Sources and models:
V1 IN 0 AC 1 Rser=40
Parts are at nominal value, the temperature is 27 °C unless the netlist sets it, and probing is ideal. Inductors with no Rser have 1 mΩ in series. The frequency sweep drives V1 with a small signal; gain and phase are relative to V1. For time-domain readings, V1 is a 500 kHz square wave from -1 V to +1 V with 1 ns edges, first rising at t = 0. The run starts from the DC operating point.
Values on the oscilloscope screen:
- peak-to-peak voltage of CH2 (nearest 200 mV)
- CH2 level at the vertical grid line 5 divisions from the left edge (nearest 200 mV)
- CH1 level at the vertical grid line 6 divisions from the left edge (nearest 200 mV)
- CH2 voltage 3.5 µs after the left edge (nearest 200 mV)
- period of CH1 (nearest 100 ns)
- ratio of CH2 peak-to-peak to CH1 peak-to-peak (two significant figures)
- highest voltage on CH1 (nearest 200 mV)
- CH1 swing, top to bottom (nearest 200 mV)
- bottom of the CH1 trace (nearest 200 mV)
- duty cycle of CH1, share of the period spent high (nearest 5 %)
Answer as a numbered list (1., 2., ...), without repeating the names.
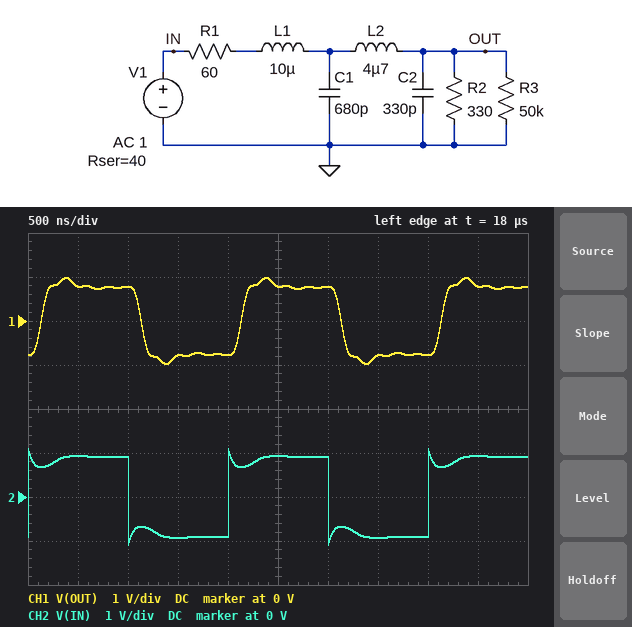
1. 2.2 V
2. 1.0 V
3. 800 mV
4. -1.0 V
5. 2.0 µs
6. 1.1
7. 1.0 V
8. 2.0 V
9. -1.0 V
10. 50 %
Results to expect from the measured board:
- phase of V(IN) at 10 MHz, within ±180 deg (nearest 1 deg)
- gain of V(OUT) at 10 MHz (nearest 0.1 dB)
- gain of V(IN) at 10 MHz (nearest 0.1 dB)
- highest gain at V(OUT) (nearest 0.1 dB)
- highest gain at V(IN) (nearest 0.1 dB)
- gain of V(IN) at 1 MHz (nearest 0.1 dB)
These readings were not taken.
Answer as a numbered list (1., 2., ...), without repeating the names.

1. 4 deg
2. -41.8 dB
3. -0.1 dB
4. -1.5 dB
5. 0 dB
6. -2.0 dB
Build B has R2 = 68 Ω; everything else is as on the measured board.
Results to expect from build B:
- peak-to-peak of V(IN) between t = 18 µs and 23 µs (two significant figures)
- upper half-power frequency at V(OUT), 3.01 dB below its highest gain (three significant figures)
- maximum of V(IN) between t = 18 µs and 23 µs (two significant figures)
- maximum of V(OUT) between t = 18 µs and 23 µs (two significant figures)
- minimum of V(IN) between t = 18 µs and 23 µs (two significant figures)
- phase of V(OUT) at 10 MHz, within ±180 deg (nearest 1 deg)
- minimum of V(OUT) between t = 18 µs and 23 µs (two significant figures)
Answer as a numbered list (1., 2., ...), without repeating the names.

1. 2.5 V
2. 3.84 MHz
3. 1.2 V
4. 440 mV
5. -1.2 V
6. 50 deg
7. -440 mV
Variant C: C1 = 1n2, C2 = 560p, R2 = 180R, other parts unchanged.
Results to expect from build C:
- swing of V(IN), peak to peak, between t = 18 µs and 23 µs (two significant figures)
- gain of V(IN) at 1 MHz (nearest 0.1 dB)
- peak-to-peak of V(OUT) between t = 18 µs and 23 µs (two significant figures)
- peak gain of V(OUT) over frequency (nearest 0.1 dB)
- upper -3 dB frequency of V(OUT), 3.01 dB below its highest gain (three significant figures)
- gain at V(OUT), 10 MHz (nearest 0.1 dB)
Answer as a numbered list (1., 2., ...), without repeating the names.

1. 2.3 V
2. -2.8 dB
3. 1.5 V
4. -3.8 dB
5. 1.78 MHz
6. -52.6 dB
